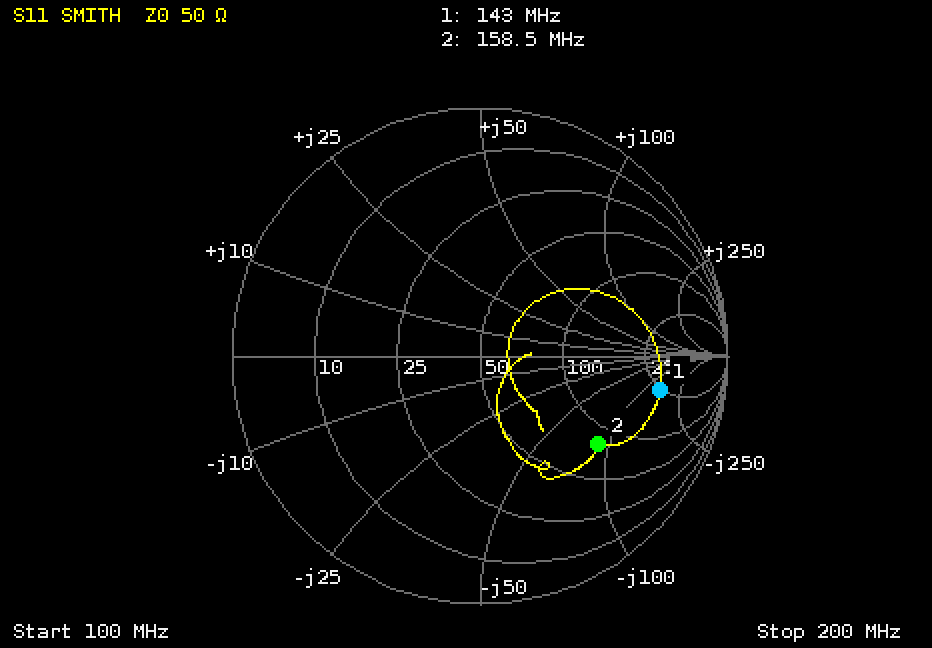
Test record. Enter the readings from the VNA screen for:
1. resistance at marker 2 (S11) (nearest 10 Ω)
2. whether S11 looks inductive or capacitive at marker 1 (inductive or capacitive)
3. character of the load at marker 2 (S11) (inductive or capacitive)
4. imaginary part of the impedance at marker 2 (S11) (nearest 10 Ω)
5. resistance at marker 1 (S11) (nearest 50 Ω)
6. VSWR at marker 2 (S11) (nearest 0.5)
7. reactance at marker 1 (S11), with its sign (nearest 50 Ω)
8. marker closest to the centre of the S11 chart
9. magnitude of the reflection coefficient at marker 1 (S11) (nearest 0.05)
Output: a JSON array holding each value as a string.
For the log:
["80 Ω", "capacitive", "capacitive", "-90 Ω", "250 Ω", "4.0", "-150 Ω", "marker 2", "0.75"]
